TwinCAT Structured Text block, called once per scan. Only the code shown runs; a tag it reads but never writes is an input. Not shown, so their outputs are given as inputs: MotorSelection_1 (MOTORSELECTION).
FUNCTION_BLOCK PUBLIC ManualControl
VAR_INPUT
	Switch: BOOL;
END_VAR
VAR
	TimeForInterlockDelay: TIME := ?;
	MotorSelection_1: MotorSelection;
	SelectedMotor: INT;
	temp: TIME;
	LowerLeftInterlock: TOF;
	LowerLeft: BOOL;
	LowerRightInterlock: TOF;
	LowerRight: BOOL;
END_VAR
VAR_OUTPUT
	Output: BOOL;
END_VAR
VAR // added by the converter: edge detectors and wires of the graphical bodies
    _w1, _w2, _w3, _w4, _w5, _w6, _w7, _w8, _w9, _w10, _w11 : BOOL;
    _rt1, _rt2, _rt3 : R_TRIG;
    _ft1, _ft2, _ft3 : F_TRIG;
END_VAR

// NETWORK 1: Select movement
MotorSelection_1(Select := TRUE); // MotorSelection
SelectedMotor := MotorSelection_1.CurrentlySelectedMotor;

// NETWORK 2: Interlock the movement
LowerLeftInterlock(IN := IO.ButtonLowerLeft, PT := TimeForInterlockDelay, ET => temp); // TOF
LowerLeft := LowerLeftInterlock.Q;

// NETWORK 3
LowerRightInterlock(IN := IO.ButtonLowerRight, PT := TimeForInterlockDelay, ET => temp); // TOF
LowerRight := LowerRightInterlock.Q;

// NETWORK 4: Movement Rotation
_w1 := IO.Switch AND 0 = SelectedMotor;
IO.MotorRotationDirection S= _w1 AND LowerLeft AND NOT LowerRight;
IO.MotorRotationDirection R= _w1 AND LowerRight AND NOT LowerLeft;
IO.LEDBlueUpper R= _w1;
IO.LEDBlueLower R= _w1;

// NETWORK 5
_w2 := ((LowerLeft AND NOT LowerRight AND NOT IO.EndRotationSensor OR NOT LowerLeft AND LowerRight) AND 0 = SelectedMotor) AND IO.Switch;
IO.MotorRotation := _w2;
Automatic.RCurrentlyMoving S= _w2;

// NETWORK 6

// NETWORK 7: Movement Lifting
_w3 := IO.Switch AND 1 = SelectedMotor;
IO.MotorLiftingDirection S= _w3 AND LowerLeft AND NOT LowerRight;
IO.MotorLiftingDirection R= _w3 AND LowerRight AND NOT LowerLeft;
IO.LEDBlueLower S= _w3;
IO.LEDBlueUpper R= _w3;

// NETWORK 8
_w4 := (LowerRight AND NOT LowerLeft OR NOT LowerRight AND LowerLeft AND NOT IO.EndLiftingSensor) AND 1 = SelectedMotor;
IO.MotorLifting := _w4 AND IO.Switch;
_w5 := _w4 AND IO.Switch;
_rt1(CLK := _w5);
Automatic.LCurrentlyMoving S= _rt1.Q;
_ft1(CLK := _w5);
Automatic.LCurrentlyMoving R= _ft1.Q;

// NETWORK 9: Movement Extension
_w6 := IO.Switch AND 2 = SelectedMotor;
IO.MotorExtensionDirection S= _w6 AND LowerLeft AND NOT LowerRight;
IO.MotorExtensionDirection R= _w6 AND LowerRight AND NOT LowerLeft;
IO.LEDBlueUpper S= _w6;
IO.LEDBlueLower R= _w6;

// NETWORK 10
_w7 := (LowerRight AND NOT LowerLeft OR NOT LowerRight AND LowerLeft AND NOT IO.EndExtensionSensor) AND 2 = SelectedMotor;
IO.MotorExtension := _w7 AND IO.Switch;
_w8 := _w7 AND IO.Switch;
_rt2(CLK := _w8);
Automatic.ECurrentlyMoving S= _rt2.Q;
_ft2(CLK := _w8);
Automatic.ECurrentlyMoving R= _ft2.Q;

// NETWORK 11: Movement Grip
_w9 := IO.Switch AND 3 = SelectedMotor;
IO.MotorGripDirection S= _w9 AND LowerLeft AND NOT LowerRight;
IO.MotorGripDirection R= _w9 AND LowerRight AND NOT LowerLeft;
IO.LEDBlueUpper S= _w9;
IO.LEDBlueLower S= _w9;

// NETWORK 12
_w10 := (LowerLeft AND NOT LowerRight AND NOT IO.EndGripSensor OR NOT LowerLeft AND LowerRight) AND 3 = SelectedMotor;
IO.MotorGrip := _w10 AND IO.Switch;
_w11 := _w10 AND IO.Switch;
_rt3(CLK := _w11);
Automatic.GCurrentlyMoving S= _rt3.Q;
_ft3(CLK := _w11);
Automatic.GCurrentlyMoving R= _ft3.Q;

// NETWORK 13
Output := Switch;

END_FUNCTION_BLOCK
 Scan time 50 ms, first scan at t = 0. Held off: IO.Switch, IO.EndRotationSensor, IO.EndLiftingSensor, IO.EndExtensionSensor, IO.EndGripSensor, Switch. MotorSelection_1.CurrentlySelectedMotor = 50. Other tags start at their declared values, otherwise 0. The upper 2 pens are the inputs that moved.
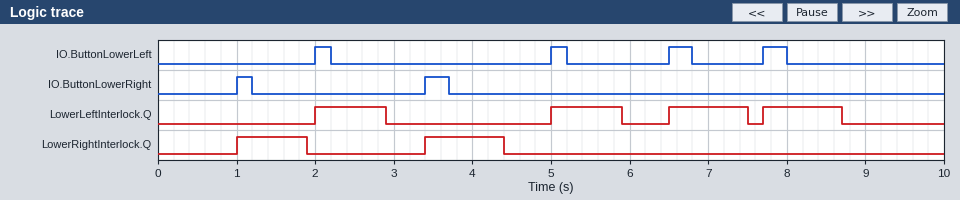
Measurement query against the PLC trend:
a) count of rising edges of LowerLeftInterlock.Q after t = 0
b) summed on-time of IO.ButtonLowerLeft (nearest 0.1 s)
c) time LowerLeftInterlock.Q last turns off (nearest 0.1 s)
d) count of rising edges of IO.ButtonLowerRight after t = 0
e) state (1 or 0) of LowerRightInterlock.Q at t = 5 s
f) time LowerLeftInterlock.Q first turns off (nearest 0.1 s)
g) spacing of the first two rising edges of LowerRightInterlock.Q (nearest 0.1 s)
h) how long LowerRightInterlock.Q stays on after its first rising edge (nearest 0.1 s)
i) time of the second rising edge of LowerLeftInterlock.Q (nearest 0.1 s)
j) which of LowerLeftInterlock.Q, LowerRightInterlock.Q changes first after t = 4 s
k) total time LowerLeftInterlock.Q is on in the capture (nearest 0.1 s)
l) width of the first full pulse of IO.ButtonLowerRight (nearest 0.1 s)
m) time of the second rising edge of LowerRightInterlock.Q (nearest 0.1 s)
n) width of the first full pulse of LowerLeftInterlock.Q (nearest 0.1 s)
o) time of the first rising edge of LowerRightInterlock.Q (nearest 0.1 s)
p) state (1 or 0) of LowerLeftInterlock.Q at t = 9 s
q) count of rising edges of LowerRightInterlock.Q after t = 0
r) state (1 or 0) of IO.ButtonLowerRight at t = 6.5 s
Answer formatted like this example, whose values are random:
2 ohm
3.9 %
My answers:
4
1.0 s
8.7 s
2
0
2.9 s
2.4 s
0.9 s
5.0 s
LowerRightInterlock.Q
3.8 s
0.2 s
3.4 s
0.9 s
1.0 s
0
2
0
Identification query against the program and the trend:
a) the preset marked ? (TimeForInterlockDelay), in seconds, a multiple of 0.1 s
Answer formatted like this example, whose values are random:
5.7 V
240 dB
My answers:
0.7 s
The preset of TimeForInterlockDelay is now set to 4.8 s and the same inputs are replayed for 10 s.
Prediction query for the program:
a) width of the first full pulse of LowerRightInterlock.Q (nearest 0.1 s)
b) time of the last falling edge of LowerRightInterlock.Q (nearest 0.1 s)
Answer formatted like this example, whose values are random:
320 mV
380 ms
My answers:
7.5 s
8.5 s
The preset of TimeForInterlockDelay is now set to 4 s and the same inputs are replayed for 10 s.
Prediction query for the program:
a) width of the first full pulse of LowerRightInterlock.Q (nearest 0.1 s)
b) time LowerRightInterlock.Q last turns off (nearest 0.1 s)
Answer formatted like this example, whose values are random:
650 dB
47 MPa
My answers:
6.7 s
7.7 s
